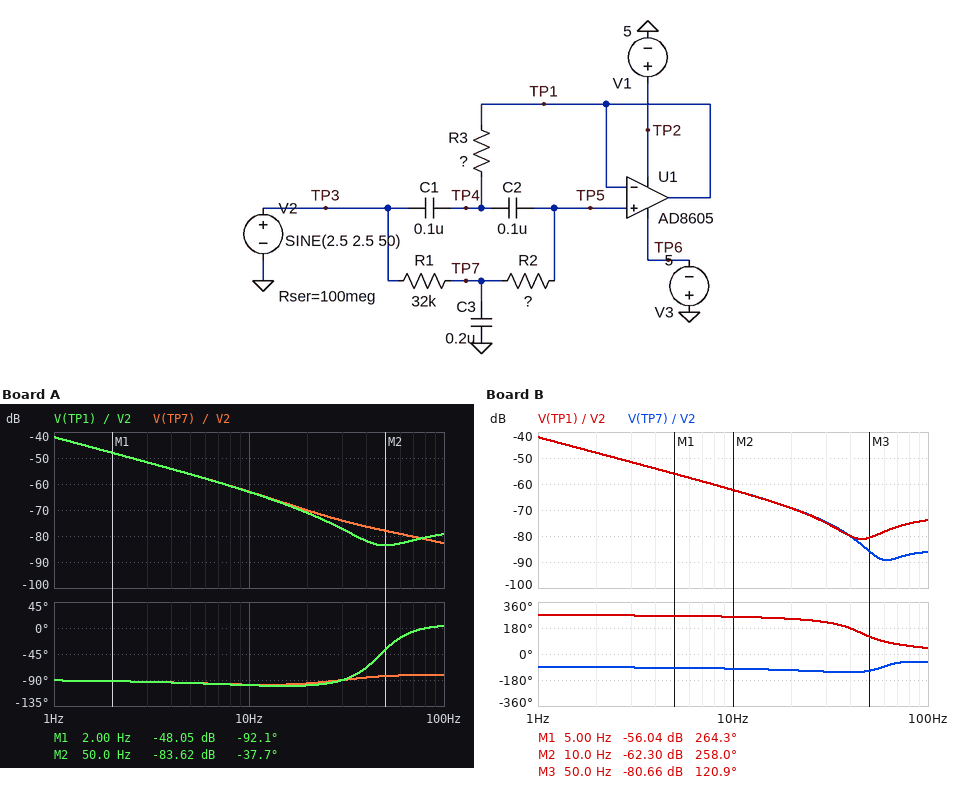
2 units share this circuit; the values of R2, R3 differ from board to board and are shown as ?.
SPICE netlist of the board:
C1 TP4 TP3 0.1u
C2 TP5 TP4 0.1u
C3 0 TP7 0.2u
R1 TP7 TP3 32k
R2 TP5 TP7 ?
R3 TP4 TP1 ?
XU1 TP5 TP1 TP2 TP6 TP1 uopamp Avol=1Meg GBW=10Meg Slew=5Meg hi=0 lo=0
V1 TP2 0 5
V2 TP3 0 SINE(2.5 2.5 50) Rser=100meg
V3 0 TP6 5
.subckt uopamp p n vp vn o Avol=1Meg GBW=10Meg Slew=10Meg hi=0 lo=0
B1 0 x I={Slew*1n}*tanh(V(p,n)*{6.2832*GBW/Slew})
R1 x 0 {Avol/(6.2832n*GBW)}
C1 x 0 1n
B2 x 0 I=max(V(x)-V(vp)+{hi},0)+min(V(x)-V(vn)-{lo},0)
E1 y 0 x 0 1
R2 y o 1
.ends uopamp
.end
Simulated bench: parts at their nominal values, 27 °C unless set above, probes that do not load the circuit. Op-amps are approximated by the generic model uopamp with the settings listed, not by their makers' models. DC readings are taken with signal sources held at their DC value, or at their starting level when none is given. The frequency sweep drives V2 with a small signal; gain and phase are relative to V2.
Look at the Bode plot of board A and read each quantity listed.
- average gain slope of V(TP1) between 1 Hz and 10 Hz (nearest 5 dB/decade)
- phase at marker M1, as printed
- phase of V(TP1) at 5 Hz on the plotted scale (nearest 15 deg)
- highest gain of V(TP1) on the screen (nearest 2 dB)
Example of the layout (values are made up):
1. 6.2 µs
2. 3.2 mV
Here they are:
1. -20 dB/decade
2. -92.1 deg
3. -90 deg
4. -42 dB
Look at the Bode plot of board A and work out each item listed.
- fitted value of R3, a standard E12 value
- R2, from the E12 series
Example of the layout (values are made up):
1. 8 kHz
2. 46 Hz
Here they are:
1. 47 kΩ
2. 27 kΩ
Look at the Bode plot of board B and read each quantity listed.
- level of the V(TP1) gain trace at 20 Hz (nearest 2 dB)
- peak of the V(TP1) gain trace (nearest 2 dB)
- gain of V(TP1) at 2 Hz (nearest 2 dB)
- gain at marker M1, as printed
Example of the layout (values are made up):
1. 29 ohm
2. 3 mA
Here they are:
1. -70 dB
2. -42 dB
3. -48 dB
4. -56.04 dB
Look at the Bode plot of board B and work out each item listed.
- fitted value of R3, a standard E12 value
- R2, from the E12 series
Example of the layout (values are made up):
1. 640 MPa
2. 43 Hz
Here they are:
1. 5.6 kΩ
2. 100 kΩ
